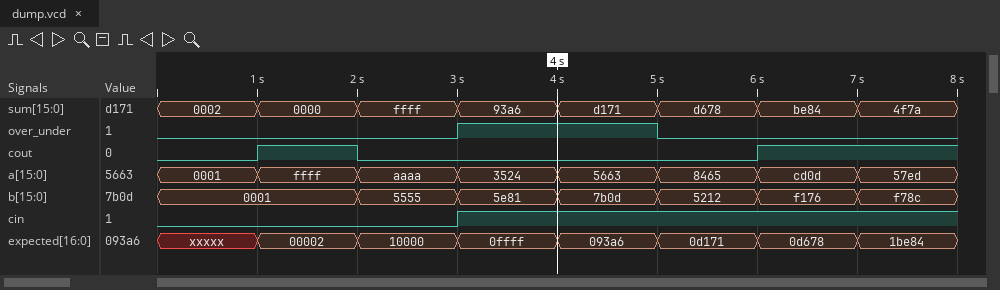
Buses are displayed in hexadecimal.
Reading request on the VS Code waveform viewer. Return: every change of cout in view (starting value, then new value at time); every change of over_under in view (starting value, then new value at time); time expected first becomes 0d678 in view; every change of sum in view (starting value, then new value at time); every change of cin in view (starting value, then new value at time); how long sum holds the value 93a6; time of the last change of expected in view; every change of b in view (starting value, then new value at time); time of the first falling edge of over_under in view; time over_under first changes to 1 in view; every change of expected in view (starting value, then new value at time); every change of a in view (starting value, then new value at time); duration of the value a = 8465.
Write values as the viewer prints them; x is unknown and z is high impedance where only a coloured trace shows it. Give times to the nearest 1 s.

0, 1 at 1 s, 0 at 2 s, 1 at 6 s
0, 1 at 3 s, 0 at 5 s
6 s
0002, 0000 at 1 s, ffff at 2 s, 93a6 at 3 s, d171 at 4 s, d678 at 5 s, be84 at 6 s, 4f7a at 7 s
0, 1 at 3 s
1 s
7 s
0001, 5555 at 2 s, 5e81 at 3 s, 7b0d at 4 s, 5212 at 5 s, f176 at 6 s, f78c at 7 s
5 s
3 s
xxxxx, 00002 at 1 s, 10000 at 2 s, 0ffff at 3 s, 093a6 at 4 s, 0d171 at 5 s, 0d678 at 6 s, 1be84 at 7 s
0001, ffff at 1 s, aaaa at 2 s, 3524 at 3 s, 5663 at 4 s, 8465 at 5 s, cd0d at 6 s, 57ed at 7 s
1 s
